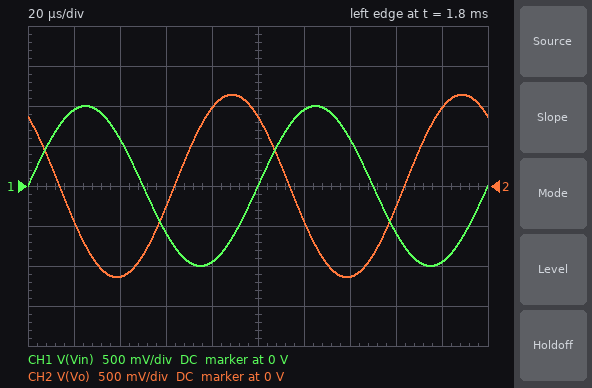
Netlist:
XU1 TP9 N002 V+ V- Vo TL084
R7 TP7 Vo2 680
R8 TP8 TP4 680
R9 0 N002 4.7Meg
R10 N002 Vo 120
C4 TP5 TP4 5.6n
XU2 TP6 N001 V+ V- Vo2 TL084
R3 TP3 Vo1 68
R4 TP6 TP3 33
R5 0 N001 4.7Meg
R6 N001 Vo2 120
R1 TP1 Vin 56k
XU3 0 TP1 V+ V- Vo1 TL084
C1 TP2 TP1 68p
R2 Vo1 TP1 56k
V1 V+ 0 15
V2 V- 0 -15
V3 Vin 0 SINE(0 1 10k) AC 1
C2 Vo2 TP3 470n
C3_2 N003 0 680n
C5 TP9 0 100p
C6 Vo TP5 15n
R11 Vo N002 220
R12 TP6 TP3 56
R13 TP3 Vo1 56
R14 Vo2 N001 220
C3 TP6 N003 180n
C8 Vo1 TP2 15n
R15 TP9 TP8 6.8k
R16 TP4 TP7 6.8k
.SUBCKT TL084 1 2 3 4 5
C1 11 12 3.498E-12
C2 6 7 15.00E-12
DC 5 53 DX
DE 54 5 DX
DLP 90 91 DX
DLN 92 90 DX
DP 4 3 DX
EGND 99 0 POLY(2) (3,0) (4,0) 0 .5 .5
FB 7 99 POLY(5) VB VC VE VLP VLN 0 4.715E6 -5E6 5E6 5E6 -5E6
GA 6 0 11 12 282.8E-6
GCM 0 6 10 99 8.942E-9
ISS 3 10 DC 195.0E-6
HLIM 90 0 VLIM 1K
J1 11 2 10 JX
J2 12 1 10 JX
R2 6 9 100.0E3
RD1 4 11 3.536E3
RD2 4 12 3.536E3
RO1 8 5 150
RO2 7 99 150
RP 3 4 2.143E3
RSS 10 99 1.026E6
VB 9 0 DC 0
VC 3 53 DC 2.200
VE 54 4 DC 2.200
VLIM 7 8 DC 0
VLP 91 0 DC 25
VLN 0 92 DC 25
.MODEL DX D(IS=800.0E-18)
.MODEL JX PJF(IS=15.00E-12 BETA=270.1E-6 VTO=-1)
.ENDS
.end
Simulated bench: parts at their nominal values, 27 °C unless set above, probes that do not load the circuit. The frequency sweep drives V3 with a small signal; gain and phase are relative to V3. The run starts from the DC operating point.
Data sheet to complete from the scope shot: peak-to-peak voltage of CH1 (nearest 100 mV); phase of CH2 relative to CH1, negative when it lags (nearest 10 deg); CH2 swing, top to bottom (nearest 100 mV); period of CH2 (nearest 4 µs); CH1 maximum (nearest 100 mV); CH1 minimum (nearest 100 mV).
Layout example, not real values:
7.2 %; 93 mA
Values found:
2.0 V; 130 deg; 2.3 V; 100 µs; 1.0 V; -1.0 V
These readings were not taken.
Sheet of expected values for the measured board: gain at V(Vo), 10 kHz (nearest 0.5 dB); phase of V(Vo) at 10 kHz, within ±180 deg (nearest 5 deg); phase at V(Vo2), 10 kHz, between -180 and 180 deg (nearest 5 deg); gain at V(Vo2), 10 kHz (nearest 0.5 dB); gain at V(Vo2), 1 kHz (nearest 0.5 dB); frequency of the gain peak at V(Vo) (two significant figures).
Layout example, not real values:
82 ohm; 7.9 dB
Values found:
1.0 dB; 130 deg; 135 deg; 0.5 dB; 0 dB; 29 kHz
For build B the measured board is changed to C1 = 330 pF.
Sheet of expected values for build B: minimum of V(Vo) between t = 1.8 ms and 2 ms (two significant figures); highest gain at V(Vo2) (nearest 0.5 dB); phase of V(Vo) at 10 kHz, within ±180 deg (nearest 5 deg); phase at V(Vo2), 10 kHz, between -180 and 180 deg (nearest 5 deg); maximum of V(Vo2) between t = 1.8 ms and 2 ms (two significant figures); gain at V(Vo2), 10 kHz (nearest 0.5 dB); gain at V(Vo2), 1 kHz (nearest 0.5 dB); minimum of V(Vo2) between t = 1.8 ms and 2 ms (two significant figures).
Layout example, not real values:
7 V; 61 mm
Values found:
-770 mV; 0 dB; 95 deg; 100 deg; 700 mV; -3.0 dB; 0 dB; -700 mV
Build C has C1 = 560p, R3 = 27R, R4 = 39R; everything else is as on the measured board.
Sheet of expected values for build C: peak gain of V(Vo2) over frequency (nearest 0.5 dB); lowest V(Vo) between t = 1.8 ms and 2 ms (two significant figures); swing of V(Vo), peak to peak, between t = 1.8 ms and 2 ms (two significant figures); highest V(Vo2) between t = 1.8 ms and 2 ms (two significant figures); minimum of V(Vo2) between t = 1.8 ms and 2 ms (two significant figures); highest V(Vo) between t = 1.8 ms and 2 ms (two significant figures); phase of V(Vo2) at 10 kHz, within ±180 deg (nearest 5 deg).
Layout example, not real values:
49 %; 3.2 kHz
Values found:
0 dB; -540 mV; 1.1 V; 490 mV; -490 mV; 540 mV; 95 deg
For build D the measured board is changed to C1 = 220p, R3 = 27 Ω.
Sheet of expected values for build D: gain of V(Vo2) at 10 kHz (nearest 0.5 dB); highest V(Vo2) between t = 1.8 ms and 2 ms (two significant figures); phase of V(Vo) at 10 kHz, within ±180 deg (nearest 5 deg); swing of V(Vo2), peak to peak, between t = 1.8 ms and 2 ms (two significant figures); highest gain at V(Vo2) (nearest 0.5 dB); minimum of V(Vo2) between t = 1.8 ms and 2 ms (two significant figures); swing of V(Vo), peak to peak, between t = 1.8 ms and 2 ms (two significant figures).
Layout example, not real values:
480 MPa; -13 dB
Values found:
-1.5 dB; 830 mV; 115 deg; 1.7 V; 0 dB; -830 mV; 1.8 V
